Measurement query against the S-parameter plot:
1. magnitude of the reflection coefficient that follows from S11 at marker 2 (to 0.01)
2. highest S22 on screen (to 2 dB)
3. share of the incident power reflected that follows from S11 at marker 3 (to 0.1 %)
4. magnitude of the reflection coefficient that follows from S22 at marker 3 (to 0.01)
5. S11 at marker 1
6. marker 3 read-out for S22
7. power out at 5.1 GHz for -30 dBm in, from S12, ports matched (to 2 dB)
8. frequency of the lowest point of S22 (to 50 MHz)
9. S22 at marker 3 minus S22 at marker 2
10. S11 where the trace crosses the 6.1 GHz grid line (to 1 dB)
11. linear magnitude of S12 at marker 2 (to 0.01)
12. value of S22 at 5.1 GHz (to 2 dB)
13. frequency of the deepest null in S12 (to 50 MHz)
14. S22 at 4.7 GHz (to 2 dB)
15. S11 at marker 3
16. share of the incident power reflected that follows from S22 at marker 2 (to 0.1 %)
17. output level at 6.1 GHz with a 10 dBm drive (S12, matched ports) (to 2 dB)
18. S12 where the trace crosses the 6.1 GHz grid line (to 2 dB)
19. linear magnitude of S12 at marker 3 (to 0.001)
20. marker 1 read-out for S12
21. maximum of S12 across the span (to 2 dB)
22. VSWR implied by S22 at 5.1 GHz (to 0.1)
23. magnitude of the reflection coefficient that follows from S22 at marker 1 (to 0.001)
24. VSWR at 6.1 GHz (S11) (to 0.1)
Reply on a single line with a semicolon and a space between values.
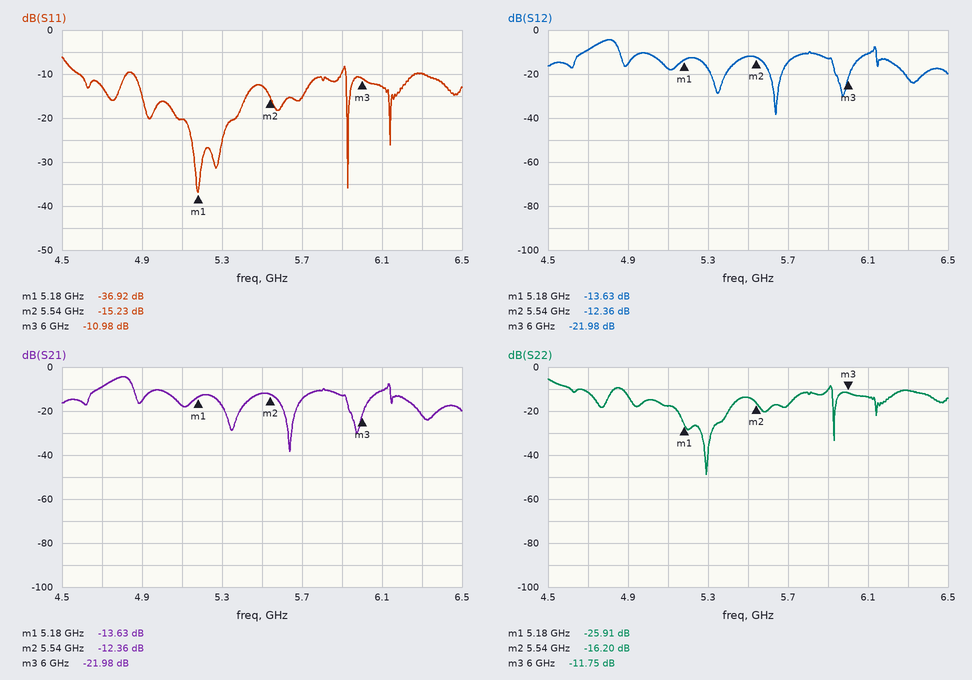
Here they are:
0.17; -6 dB; 8.0 %; 0.26; -36.92 dB; -11.75 dB; -48 dBm; 5.30 GHz; 4.45 dB; -13 dB; 0.24; -18 dB; 5.65 GHz; -12 dB; -10.98 dB; 2.4 %; 0 dBm; -10 dB; 0.080; -13.63 dB; -4 dB; 1.3; 0.051; 1.6
